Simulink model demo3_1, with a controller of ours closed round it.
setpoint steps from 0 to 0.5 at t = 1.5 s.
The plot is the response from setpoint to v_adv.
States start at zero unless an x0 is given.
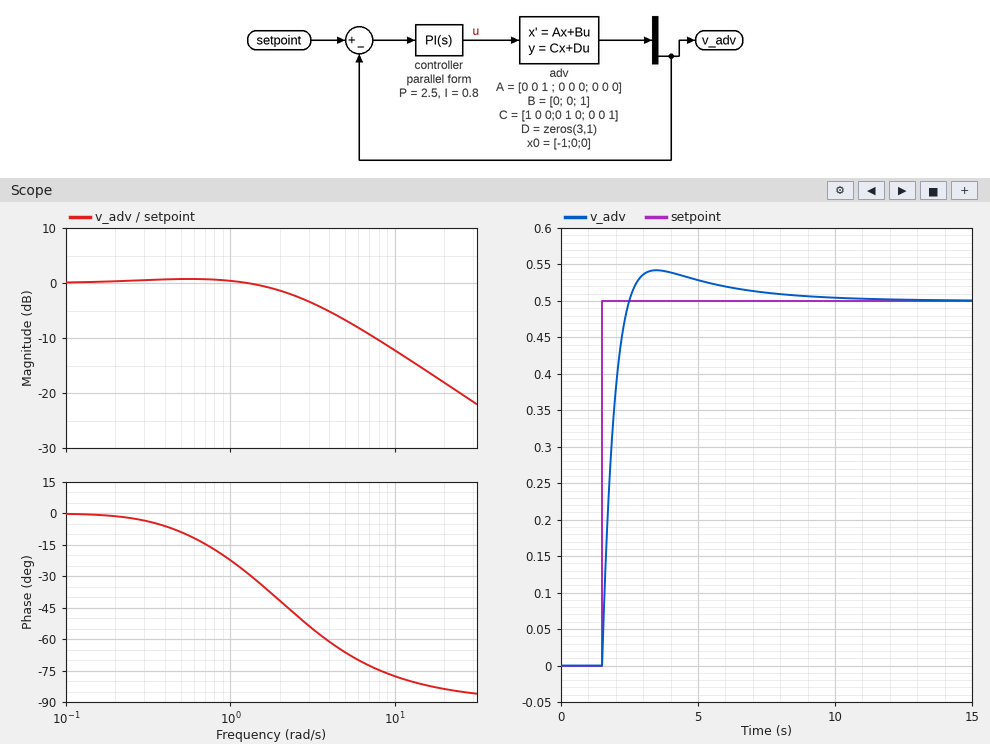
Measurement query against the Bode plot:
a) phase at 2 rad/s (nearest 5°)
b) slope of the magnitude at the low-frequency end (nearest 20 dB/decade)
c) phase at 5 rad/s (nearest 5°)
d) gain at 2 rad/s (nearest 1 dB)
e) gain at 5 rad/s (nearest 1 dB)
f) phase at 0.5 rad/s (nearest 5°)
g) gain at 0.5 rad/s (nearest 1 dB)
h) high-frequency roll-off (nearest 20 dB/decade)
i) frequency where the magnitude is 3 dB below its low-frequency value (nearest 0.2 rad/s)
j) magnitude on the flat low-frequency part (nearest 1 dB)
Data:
-40°
0 dB/decade
-65°
-1 dB
-7 dB
-10°
1 dB
-20 dB/decade
2.8 rad/s
0 dB
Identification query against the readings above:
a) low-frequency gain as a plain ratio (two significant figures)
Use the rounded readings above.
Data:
1.0
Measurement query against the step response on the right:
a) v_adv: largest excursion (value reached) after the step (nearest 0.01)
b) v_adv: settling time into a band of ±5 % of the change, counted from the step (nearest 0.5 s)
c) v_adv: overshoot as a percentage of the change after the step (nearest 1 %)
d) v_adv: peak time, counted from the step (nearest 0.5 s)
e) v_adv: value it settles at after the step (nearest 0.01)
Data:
0.54
4.0 s
8 %
2.0 s
0.50
